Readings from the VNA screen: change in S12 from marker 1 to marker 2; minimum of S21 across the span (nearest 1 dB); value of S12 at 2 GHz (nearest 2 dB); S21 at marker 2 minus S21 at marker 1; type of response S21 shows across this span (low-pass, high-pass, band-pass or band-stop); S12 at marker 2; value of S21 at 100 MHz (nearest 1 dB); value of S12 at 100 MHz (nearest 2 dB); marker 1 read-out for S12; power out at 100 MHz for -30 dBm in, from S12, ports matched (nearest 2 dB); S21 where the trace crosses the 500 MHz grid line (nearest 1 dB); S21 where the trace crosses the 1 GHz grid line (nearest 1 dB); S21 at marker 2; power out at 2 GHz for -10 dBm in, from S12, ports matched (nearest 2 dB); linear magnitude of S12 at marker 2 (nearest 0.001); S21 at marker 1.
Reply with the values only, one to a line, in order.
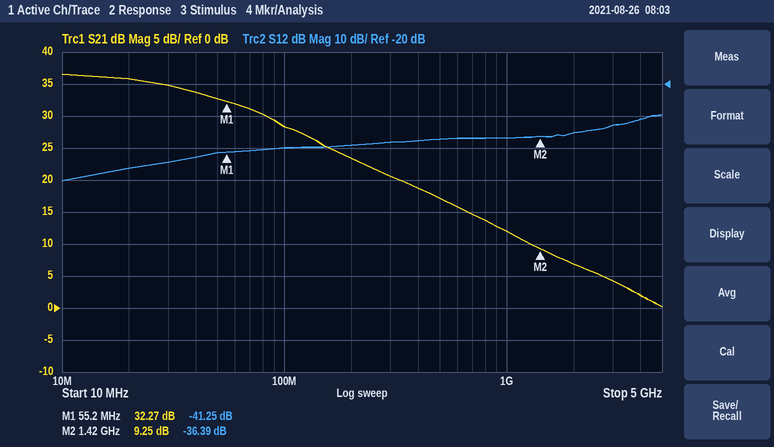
4.86 dB
0 dB
-36 dB
-23.02 dB
low-pass
-36.39 dB
28 dB
-40 dB
-41.25 dB
-70 dBm
17 dB
12 dB
9.25 dB
-46 dBm
0.015
32.27 dB
